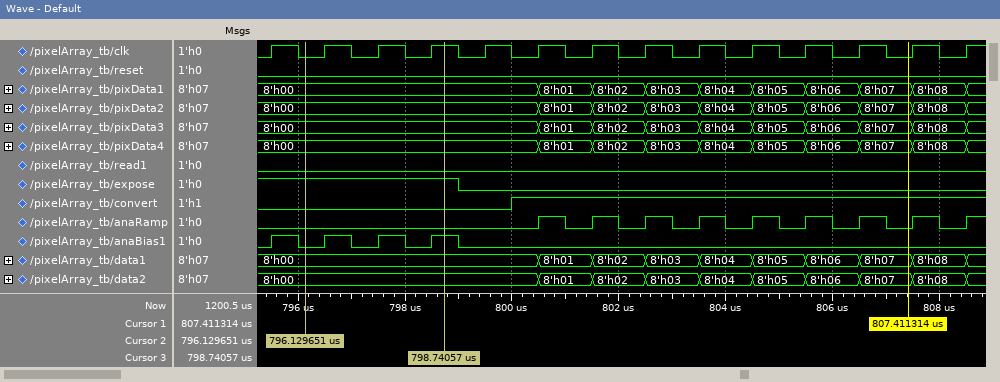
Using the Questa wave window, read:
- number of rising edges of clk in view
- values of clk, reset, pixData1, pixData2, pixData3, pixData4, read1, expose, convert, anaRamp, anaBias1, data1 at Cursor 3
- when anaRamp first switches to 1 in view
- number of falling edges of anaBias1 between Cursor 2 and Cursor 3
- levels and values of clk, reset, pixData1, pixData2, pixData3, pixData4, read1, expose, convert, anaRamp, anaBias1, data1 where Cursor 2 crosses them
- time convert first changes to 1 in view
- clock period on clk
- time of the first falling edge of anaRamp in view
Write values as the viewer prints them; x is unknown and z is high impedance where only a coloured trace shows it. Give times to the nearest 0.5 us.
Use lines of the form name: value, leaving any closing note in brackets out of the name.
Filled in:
number of rising edges of clk in view: 14
values of clk, reset, pixData1, pixData2, pixData3, pixData4, read1, expose, convert, anaRamp, anaBias1, data1 at Cursor 3: clk=1, reset=0, pixData1=8'h00, pixData2=8'h00, pixData3=8'h00, pixData4=8'h00, read1=0, expose=1, convert=0, anaRamp=0, anaBias1=1, data1=8'h00
when anaRamp first switches to 1 in view: 800.5 us
number of falling edges of anaBias1 between Cursor 2 and Cursor 3: 2
levels and values of clk, reset, pixData1, pixData2, pixData3, pixData4, read1, expose, convert, anaRamp, anaBias1, data1 where Cursor 2 crosses them: clk=0, reset=0, pixData1=8'h00, pixData2=8'h00, pixData3=8'h00, pixData4=8'h00, read1=0, expose=1, convert=0, anaRamp=0, anaBias1=0, data1=8'h00
time convert first changes to 1 in view: 800 us
clock period on clk: 1 us
time of the first falling edge of anaRamp in view: 801 us
